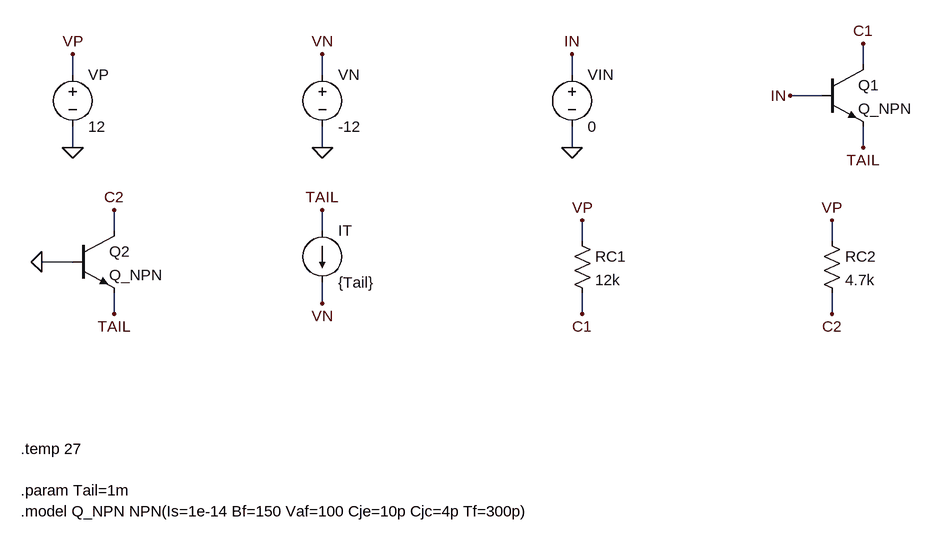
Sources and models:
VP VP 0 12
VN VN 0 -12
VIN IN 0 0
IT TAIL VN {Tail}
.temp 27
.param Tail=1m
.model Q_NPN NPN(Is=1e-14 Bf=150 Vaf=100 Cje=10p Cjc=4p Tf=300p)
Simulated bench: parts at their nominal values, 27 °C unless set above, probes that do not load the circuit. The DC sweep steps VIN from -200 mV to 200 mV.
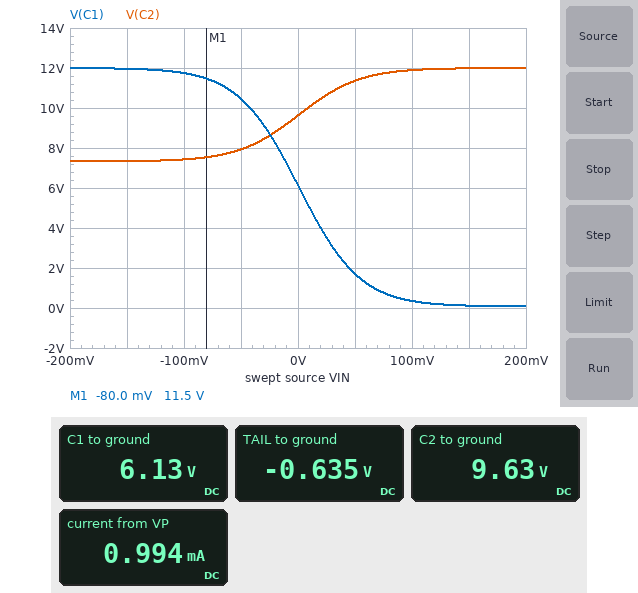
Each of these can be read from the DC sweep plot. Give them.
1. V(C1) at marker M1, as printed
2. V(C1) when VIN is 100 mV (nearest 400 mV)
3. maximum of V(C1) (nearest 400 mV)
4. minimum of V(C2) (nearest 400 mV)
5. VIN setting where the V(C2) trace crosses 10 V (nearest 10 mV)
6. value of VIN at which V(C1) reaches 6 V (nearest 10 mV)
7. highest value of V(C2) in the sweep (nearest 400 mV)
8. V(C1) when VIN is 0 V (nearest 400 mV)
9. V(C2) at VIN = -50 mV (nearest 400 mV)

11.5 V
400 mV
12.0 V
7.2 V
10 mV
0 V
12.0 V
6.0 V
8.0 V
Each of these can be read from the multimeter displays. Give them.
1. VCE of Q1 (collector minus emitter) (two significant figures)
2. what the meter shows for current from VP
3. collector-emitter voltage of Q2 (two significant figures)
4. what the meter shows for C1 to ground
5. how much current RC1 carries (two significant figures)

6.8 V
0.994 mA
10 V
6.13 V
490 µA
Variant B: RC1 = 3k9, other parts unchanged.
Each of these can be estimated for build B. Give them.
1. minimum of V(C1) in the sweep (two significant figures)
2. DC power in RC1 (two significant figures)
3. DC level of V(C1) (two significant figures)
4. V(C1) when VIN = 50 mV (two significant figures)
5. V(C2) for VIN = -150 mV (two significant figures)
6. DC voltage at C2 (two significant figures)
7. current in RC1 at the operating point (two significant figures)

8.1 V
970 µW
10 V
8.6 V
7.3 V
9.7 V
500 µA
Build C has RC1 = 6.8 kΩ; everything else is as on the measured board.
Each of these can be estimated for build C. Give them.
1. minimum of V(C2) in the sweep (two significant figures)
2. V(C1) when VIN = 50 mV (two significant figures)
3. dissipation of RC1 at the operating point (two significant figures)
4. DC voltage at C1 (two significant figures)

7.3 V
6.1 V
1.7 mW
8.6 V
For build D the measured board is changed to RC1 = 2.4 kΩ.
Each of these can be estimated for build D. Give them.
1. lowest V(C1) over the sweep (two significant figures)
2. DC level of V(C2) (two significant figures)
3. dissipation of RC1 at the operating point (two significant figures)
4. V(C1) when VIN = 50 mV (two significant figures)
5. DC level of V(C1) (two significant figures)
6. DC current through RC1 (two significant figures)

9.6 V
9.7 V
600 µW
9.9 V
11 V
500 µA
